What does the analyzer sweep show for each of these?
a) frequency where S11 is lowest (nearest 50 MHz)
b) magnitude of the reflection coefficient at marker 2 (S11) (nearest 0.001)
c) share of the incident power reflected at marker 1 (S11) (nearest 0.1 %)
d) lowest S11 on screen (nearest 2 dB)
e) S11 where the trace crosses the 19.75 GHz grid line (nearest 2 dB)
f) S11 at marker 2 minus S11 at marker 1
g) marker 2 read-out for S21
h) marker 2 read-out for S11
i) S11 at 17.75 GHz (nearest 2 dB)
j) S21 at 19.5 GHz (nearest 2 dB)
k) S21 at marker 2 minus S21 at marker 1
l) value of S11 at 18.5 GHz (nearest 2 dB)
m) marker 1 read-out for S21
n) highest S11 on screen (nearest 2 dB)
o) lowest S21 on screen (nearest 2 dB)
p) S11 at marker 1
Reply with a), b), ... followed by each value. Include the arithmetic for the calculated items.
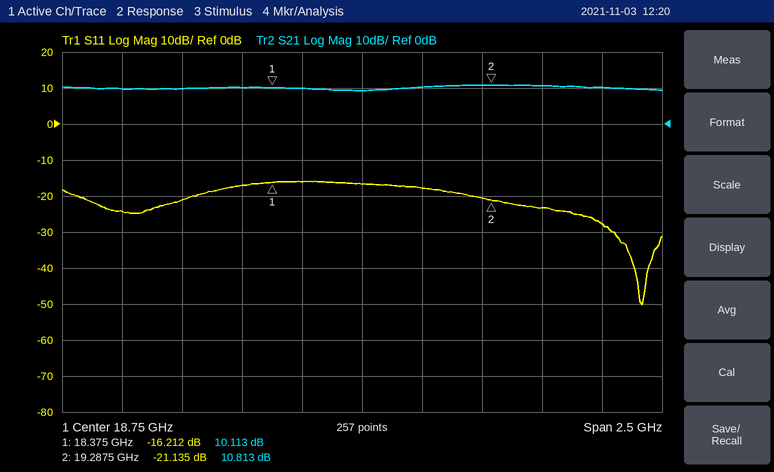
a) 19.90 GHz
b) 10^(-21.135/20) ≈ 0.088
c) 10^(-16.212/10) ≈ 2.4 %
d) -50 dB
e) -28 dB
f) -21.135 − (-16.212) = -4.923 dB
g) 10.813 dB
h) -21.135 dB
i) -24 dB
j) 10 dB
k) 10.813 − (10.113) = 0.700 dB
l) -16 dB
m) 10.113 dB
n) -16 dB
o) 10 dB
p) -16.212 dB
